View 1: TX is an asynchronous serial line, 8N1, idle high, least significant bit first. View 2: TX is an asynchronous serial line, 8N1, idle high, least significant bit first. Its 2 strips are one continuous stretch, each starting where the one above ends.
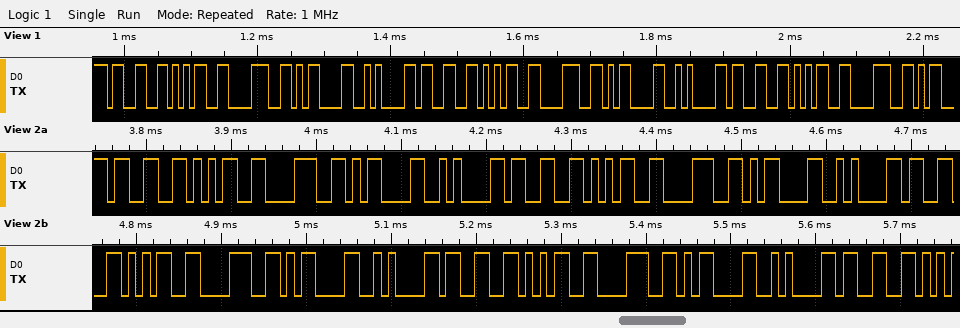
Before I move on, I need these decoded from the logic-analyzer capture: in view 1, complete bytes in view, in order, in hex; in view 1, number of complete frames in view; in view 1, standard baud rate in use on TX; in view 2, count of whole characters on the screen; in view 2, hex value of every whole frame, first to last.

33 35 38 0D 0A 33 35 38 0D 0A 33 35 38
13
115200 baud
21
0x33 0x35 0x38 0x0D 0x0A 0x33 0x35 0x38 0x0D 0x0A 0x33 0x35 0x38 0x0D 0x0A 0x33 0x35 0x38 0x0D 0x0A 0x33
